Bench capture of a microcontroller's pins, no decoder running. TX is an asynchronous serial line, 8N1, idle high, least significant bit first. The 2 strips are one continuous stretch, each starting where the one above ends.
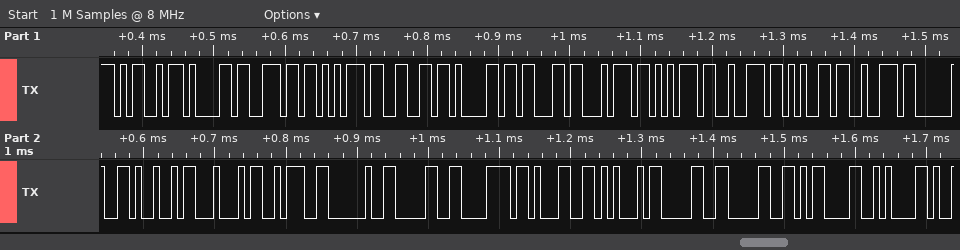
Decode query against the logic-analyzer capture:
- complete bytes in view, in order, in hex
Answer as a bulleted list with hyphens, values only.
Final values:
- 0x4D 0x61 0x6E 0x75 0x66 0x61 0x63 0x74 0x75 0x72 0x65 0x72 0x20 0x49 0x44 0x3A 0x20 0x30 0x78 0x31 0x45 0x30 0x30 0x0D 0x0A
